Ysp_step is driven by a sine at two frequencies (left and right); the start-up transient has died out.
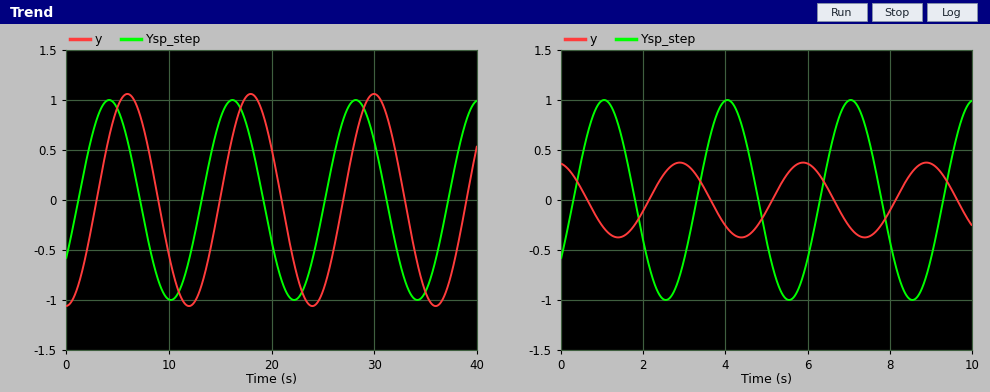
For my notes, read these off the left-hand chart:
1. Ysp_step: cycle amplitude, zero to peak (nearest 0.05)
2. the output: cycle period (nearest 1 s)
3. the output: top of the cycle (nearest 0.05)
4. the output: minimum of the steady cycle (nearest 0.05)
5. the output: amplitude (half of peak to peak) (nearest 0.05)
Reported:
1.00
12 s
1.05
-1.05
1.05
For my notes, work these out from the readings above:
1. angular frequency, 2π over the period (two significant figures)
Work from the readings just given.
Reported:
0.52 rad/s
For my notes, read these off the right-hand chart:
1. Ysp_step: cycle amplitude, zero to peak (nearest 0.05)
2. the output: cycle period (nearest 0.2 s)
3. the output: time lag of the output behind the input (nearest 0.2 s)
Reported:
1.00
3.0 s
1.8 s
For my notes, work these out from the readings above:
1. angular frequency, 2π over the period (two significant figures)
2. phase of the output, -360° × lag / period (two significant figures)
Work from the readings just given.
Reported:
2.1 rad/s
-220°
